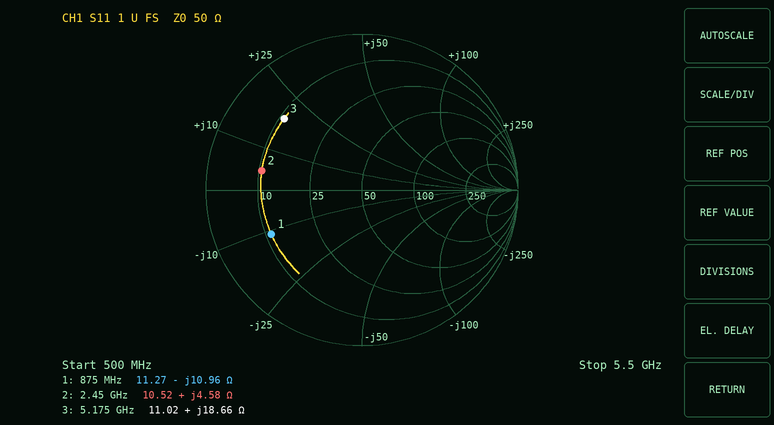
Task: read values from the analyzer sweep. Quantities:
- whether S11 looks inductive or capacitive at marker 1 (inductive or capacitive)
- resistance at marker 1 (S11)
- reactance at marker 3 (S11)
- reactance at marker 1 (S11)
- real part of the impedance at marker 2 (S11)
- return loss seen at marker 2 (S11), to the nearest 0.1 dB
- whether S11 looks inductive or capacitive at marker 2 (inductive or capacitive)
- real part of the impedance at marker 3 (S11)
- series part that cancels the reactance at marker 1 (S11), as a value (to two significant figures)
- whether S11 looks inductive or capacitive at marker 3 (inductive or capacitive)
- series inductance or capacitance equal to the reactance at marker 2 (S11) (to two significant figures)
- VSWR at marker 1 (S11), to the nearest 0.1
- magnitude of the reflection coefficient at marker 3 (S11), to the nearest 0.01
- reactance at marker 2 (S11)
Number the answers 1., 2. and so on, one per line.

1. capacitive
2. 11.27 Ω
3. +18.66 Ω
4. -10.96 Ω
5. 10.52 Ω
6. 3.7 dB
7. inductive
8. 11.02 Ω
9. 2.0 nH
10. inductive
11. 300 pH
12. 4.7
13. 0.68
14. +4.58 Ω
